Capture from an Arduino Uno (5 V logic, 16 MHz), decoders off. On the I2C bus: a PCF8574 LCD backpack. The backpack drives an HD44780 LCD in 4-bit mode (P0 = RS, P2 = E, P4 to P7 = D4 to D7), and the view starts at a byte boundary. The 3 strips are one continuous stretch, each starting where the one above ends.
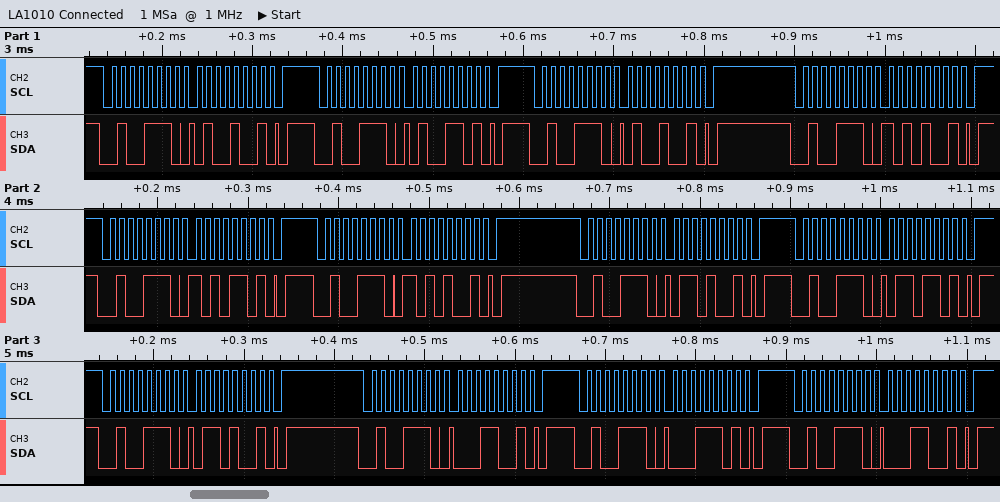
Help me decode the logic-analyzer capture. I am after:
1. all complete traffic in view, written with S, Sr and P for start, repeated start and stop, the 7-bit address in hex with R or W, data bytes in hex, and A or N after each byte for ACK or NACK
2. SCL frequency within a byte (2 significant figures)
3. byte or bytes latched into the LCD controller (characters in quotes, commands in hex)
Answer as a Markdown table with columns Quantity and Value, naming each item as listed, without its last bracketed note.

| Quantity | Value |
|---|---|
| all complete traffic in view, written with S, Sr and P for start, repeated start and stop, the 7-bit address in hex with R or W, data bytes in hex, and A or N after each byte for ACK or NACK | S 27W A 49 A P S 27W A 4D A P S 27W A 49 A P S 27W A A9 A P S 27W A AD A P S 27W A A9 A P S 27W A 69 A P S 27W A 6D A P S 27W A 69 A P S 27W A 19 A P S 27W A 1D A P S 27W A 19 A P |
| SCL frequency within a byte | 100 kHz |
| byte or bytes latched into the LCD controller | 'J' 'a' |
